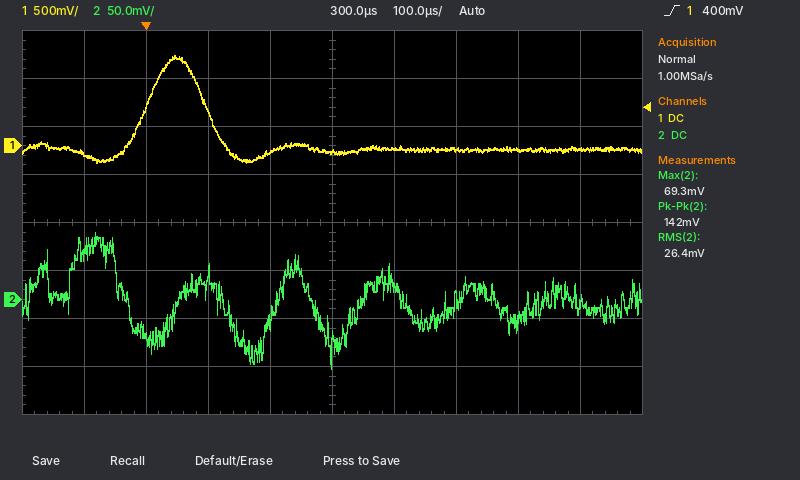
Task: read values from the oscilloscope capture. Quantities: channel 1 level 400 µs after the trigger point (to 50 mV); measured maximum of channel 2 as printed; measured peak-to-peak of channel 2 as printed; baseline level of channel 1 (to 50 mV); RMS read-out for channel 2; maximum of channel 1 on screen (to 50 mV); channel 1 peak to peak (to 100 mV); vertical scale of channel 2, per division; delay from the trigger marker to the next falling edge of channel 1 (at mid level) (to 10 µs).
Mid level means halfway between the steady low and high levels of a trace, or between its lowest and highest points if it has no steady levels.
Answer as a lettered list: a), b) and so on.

a) -50 mV
b) 69.3 mV
c) 142 mV
d) -50 mV
e) 26.4 mV
f) 950 mV
g) 1.10 V
h) 50 mV
i) 100 µs
